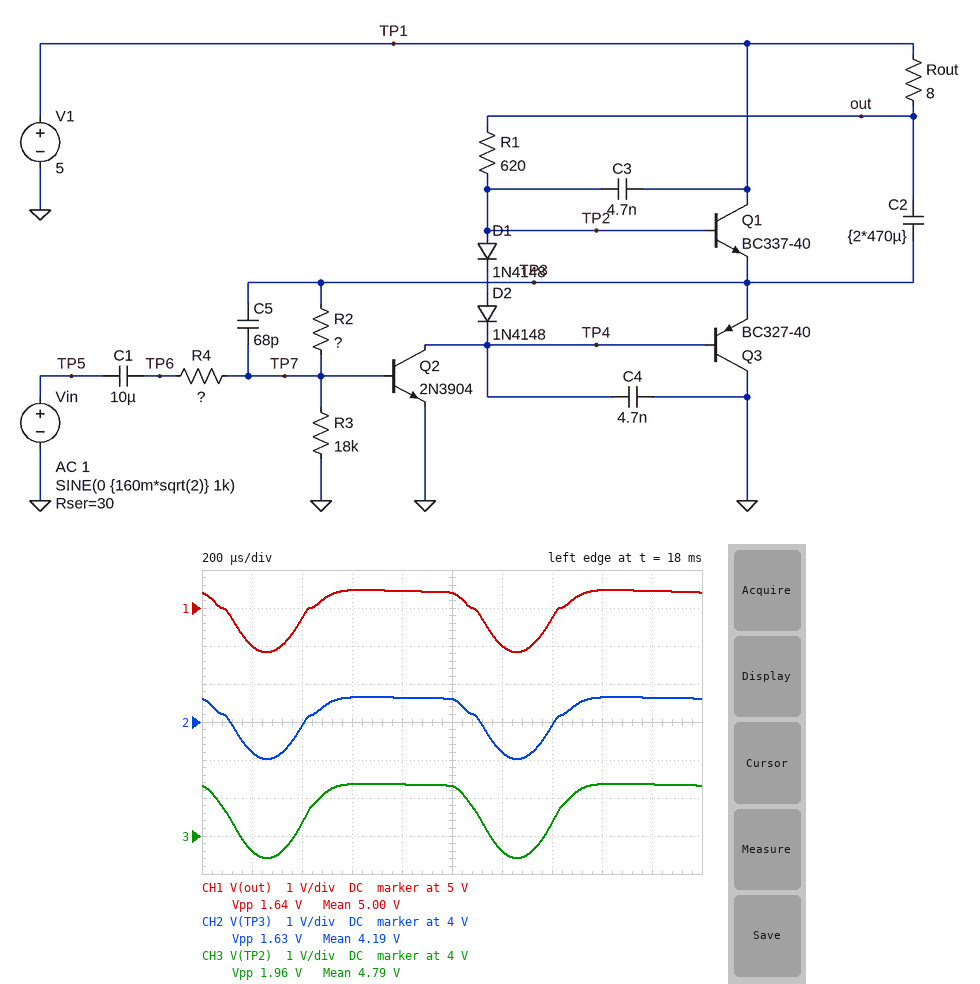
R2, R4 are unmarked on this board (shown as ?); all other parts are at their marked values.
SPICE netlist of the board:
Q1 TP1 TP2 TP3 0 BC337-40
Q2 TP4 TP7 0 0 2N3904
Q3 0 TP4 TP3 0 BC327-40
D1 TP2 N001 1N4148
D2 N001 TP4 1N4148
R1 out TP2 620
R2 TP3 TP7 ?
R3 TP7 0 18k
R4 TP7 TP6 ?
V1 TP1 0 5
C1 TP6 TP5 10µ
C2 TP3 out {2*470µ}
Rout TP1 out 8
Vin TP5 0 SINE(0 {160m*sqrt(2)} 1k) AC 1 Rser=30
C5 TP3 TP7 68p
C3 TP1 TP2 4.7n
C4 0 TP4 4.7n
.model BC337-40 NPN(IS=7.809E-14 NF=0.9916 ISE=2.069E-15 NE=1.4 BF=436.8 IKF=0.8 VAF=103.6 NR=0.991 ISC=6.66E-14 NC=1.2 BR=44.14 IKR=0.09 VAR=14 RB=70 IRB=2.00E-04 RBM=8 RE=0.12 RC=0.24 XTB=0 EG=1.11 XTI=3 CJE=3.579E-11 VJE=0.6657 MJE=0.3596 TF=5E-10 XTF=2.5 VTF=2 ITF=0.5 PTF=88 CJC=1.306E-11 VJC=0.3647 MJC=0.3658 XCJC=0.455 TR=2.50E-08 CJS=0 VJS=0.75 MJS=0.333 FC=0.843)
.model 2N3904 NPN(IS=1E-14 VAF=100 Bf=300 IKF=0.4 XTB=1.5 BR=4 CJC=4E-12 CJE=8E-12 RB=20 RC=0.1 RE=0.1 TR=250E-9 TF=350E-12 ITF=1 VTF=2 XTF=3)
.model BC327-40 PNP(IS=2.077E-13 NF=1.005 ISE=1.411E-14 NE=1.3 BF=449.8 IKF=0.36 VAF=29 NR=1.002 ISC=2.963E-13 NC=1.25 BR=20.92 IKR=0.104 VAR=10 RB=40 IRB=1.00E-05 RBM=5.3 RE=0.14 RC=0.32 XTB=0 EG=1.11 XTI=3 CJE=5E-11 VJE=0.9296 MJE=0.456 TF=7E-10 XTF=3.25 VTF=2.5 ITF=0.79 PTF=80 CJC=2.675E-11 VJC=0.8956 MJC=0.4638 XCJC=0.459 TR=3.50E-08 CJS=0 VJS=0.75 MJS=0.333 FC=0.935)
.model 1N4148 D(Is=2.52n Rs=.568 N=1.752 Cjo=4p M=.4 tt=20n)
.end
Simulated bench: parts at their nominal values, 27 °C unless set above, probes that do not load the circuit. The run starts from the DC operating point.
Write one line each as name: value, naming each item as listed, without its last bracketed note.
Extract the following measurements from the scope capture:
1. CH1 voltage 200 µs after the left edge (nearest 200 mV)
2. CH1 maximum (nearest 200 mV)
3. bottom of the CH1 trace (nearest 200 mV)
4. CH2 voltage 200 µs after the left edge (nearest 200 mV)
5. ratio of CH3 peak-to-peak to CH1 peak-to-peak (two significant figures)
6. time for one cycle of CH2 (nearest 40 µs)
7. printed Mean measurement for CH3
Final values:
CH1 voltage 200 µs after the left edge: 4.0 V
CH1 maximum: 5.4 V
bottom of the CH1 trace: 3.8 V
CH2 voltage 200 µs after the left edge: 3.2 V
ratio of CH3 peak-to-peak to CH1 peak-to-peak: 1.2
time for one cycle of CH2: 1.00 ms
printed Mean measurement for CH3: 4.79 V
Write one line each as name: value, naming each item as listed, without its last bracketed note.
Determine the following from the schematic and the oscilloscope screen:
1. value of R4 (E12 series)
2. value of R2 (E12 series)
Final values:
value of R4: 6.8 kΩ
value of R2: 120 kΩ
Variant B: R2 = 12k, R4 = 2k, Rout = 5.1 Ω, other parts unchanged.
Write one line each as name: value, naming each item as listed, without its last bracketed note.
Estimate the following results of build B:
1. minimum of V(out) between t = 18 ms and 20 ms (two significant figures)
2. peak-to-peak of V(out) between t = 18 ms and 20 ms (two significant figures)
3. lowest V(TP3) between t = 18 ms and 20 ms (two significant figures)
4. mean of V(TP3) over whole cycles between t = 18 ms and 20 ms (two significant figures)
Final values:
minimum of V(out) between t = 18 ms and 20 ms: 4.3 V
peak-to-peak of V(out) between t = 18 ms and 20 ms: 1.8 V
lowest V(TP3) between t = 18 ms and 20 ms: 820 mV
mean of V(TP3) over whole cycles between t = 18 ms and 20 ms: 1.5 V
